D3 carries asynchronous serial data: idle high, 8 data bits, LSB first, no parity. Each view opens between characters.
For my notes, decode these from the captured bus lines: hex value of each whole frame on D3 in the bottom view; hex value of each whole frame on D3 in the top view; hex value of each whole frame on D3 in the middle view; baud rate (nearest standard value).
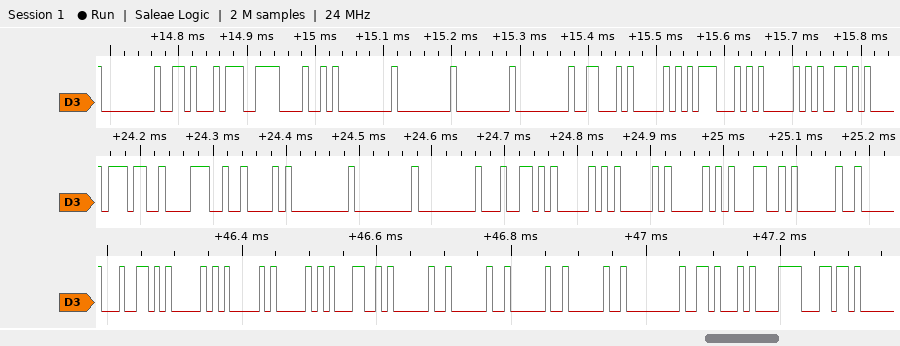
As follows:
64, 41, 41, 50, 4C, 20, 20, 20, 20, 00, 16, E1, 6C
00, 16, E7, 48, 00, 00, 00, 00, 46, 50, 47, 41, 59
37, 38, 42, 00, 00, 00, 64, 41, 41, 50, 4C, 20
115200 baud
